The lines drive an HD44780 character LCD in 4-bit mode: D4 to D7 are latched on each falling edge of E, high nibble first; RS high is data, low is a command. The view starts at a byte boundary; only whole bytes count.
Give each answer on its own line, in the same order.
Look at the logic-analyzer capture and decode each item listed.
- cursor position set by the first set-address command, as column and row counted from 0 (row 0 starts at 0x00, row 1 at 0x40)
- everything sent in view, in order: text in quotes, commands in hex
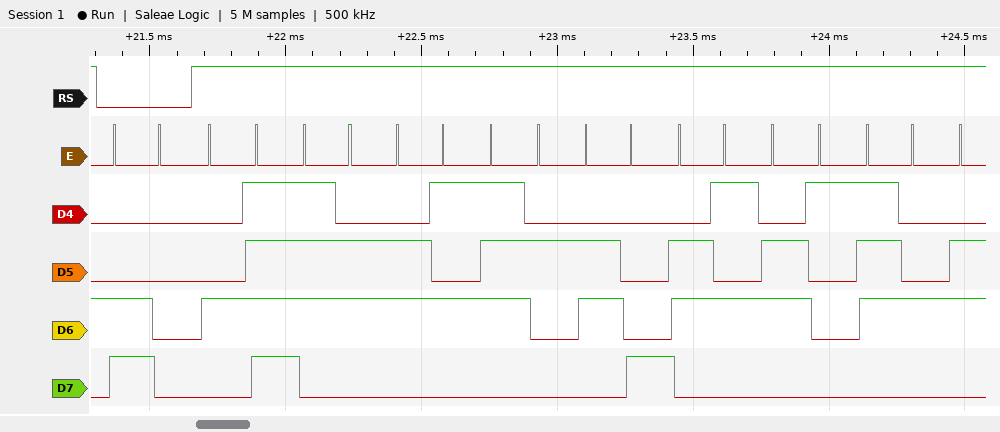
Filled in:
column 0, row 1
0xC0 "Overheat"
